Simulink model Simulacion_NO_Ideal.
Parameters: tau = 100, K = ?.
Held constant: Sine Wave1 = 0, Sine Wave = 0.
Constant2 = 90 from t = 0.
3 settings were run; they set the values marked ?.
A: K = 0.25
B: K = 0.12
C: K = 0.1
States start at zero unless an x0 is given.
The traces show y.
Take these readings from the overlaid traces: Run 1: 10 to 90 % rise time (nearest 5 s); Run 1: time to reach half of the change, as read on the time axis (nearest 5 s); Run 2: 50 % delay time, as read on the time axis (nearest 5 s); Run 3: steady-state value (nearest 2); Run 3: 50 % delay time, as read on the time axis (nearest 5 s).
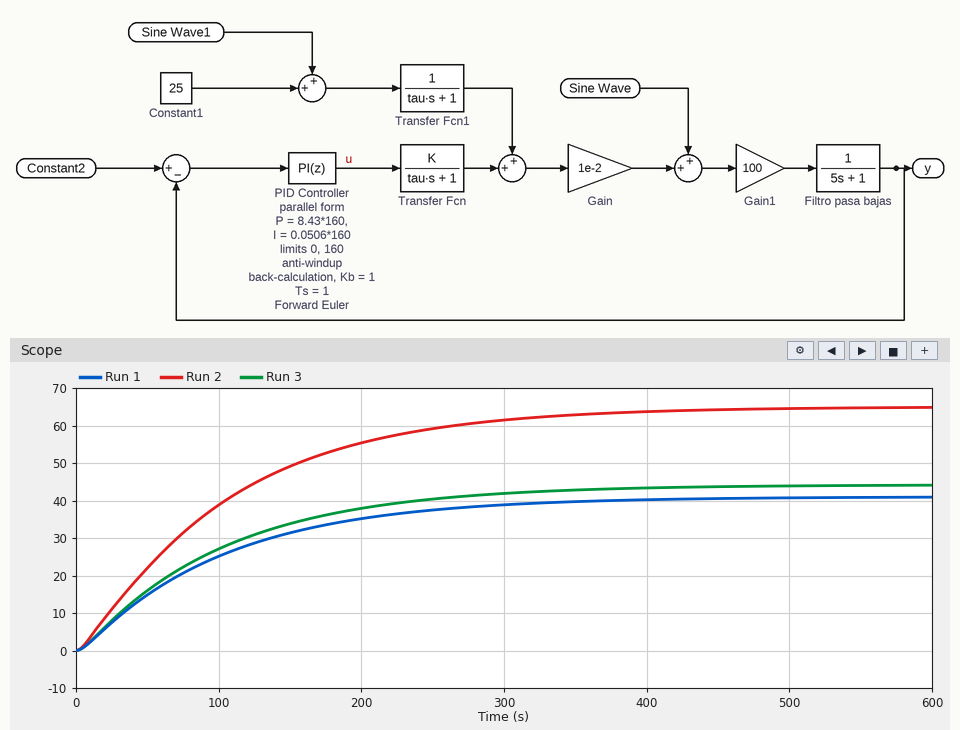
220 s
75 s
80 s
44
75 s
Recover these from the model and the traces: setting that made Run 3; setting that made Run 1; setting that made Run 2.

B
C
A
